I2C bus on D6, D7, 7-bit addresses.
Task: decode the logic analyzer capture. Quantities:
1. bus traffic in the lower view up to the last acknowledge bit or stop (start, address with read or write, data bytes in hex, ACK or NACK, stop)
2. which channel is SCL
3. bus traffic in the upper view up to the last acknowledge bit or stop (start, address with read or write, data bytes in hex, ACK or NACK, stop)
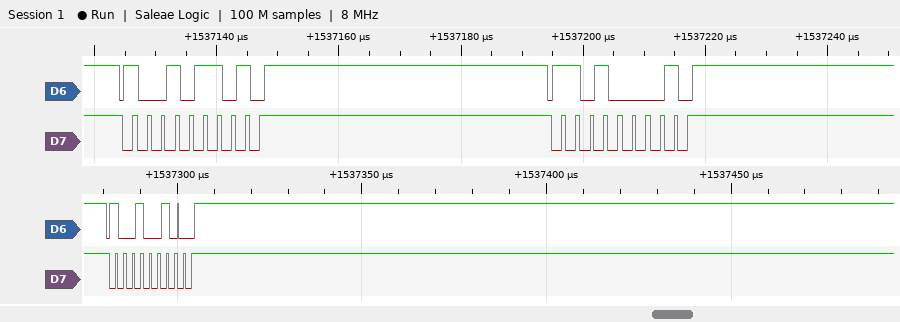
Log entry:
start, address 49 write ACK, stop
D7
start, address 4B write NACK, stop, start, address 68 write NACK, stop
